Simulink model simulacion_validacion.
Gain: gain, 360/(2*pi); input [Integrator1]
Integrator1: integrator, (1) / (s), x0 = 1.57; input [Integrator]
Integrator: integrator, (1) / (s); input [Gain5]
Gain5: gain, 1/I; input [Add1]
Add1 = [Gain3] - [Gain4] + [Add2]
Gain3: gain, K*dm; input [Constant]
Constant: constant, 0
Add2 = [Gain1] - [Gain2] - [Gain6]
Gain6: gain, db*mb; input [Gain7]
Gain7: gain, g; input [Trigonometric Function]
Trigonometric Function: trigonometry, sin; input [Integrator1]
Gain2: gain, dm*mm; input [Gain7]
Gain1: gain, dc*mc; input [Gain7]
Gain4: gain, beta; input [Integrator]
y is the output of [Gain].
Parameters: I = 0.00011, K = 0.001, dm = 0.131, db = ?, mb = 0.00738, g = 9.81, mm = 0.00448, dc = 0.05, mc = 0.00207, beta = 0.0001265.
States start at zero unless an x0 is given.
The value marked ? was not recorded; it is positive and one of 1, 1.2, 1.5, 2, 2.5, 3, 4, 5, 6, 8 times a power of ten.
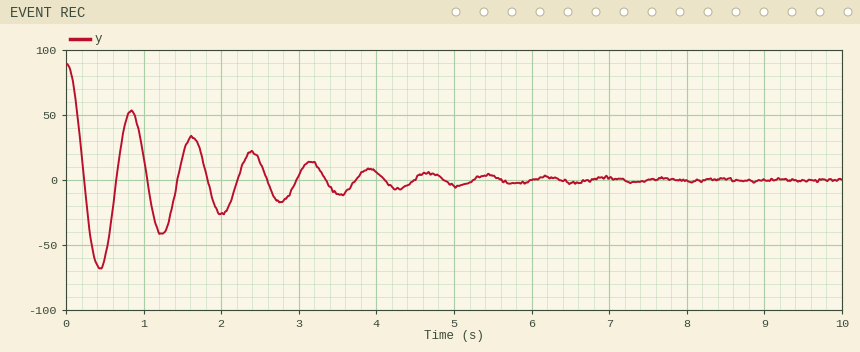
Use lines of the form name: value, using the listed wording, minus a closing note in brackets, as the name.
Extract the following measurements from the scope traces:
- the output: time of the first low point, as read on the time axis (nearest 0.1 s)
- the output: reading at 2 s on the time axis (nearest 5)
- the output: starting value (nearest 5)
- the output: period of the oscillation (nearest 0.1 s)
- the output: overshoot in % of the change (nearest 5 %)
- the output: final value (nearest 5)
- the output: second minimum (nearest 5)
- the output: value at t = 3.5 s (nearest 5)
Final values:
the output: time of the first low point, as read on the time axis: 0.4 s
the output: reading at 2 s on the time axis: -25
the output: starting value: 90
the output: period of the oscillation: 0.8 s
the output: overshoot in % of the change: 75 %
the output: final value: 0
the output: second minimum: -40
the output: value at t = 3.5 s: -10
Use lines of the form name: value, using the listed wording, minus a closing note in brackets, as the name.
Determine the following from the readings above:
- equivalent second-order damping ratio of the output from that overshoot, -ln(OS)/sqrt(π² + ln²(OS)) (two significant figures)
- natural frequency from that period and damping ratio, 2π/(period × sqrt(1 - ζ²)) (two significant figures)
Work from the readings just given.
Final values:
equivalent second-order damping ratio of the output from that overshoot, -ln(OS)/sqrt(π² + ln²(OS)): 0.091
natural frequency from that period and damping ratio, 2π/(period × sqrt(1 - ζ²)): 7.9 rad/s
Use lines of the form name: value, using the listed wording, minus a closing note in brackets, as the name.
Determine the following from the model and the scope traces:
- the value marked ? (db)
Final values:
the value marked ?: 0.04
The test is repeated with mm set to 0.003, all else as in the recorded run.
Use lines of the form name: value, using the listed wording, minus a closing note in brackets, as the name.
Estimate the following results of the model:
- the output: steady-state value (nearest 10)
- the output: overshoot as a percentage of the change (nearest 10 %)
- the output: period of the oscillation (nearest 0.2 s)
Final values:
the output: steady-state value: 0
the output: overshoot as a percentage of the change: 70 %
the output: period of the oscillation: 1.0 s
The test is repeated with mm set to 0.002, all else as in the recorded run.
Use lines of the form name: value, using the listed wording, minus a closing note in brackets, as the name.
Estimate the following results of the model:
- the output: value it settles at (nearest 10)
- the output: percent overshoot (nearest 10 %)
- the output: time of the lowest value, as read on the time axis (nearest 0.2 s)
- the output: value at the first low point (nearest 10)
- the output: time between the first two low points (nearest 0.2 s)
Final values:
the output: value it settles at: 0
the output: percent overshoot: 70 %
the output: time of the lowest value, as read on the time axis: 0.6 s
the output: value at the first low point: -60
the output: time between the first two low points: 1.0 s
